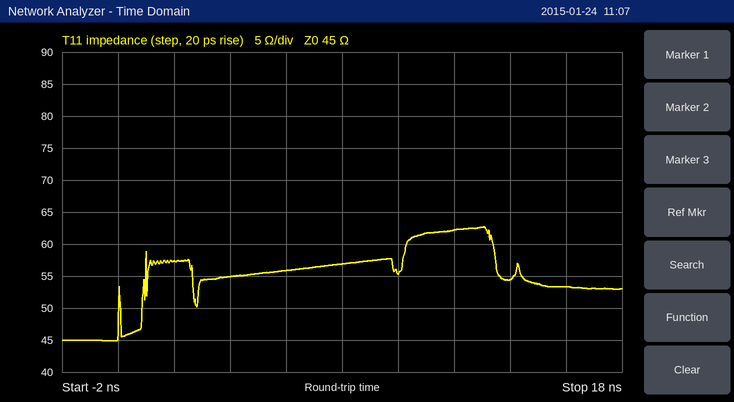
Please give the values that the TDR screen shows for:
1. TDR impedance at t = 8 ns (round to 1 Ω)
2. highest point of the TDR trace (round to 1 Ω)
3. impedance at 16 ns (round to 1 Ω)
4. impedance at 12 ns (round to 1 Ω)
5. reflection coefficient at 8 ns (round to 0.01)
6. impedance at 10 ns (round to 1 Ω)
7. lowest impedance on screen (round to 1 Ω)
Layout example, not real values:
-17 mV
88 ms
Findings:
57 Ω
63 Ω
53 Ω
62 Ω
+0.12
55 Ω
45 Ω
